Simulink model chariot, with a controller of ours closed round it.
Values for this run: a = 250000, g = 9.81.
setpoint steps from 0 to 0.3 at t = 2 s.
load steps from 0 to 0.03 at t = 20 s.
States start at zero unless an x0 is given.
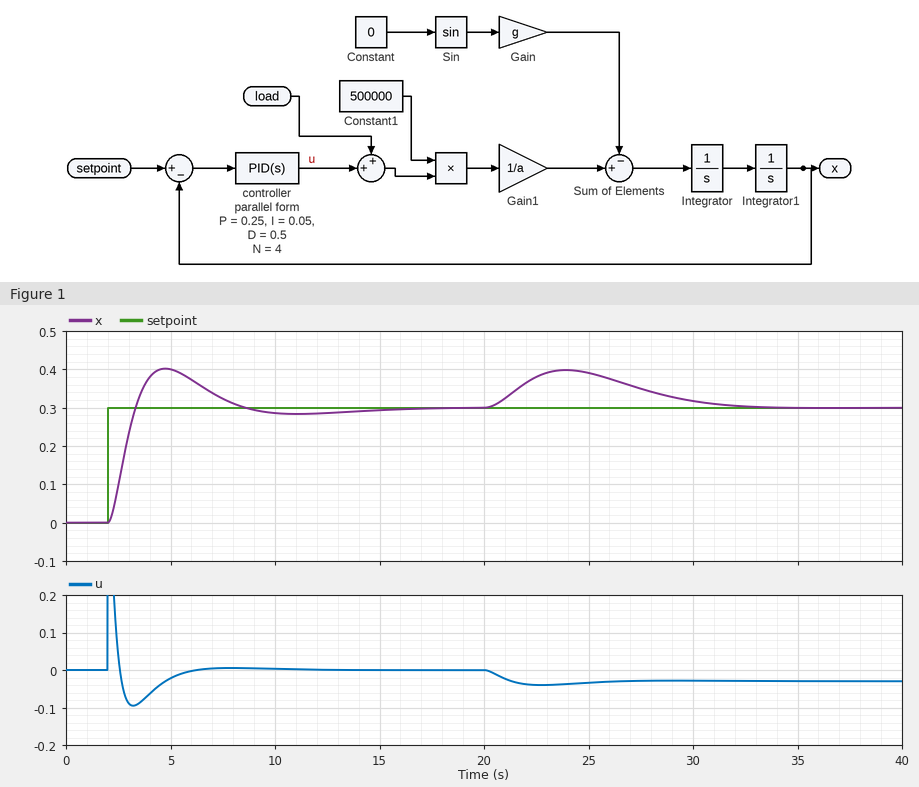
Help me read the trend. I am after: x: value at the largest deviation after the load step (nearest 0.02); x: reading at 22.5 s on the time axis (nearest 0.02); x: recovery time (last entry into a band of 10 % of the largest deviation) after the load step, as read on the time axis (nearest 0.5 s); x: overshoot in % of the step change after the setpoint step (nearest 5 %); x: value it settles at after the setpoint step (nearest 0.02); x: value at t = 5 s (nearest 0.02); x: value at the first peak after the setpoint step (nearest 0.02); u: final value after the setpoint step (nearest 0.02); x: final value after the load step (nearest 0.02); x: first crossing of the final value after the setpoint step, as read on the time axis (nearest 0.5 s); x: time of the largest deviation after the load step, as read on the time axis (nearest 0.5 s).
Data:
0.40
0.38
31.0 s
35 %
0.30
0.40
0.40
0.00
0.30
3.5 s
24.0 s
